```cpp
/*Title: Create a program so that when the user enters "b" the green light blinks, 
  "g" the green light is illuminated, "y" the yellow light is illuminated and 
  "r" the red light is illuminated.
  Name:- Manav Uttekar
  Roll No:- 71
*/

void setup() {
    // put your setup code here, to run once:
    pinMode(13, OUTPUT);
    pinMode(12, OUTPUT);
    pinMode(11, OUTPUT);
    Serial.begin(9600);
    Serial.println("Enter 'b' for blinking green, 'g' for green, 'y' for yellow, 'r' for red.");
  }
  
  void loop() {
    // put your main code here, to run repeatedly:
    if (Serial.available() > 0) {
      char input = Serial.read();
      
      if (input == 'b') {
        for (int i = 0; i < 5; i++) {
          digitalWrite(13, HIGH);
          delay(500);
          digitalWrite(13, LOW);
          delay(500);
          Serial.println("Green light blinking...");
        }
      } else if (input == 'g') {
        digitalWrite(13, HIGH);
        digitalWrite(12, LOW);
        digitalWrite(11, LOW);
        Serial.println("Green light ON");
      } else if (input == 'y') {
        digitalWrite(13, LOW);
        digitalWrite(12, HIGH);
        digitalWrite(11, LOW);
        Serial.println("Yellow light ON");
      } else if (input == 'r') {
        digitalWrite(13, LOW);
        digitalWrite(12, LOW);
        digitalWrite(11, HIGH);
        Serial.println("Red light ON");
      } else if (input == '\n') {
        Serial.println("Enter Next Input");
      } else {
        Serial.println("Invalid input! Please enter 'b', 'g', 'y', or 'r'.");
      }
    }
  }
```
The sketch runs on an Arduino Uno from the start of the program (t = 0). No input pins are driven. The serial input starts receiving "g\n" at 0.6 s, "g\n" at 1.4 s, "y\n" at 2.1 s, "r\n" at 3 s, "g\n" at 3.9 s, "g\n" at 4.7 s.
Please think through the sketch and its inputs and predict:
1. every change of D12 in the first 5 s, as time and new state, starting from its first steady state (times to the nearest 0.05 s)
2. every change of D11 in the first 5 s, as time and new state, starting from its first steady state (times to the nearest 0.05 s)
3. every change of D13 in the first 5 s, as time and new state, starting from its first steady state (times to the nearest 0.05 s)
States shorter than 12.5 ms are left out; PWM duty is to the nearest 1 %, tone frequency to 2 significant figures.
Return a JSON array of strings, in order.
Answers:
["0 s low; 2.1 s high; 3 s low", "0 s low; 3 s high; 3.9 s low", "0 s low; 0.6 s high; 2.1 s low; 3.9 s high"]
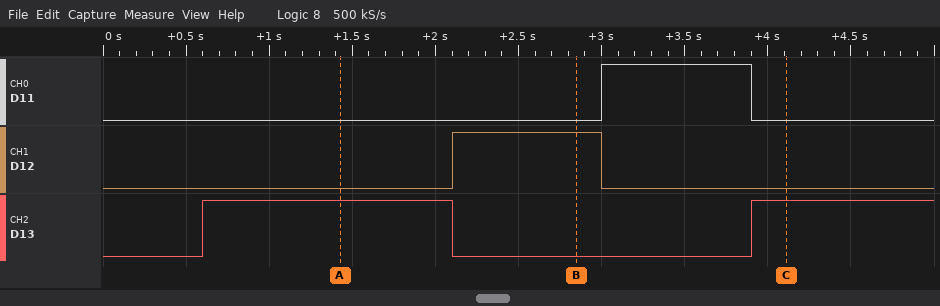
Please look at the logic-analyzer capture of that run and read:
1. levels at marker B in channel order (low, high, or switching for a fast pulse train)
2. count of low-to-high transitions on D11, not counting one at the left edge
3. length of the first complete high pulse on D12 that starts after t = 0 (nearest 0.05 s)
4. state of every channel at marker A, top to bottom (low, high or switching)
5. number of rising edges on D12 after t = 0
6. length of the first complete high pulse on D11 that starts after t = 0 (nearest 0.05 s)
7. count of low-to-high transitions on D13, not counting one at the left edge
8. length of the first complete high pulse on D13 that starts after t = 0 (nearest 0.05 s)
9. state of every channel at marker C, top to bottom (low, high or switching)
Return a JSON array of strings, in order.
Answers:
["D11 low, D12 high, D13 low", "1", "0.90 s", "D11 low, D12 low, D13 high", "1", "0.90 s", "2", "1.50 s", "D11 low, D12 low, D13 high"]
